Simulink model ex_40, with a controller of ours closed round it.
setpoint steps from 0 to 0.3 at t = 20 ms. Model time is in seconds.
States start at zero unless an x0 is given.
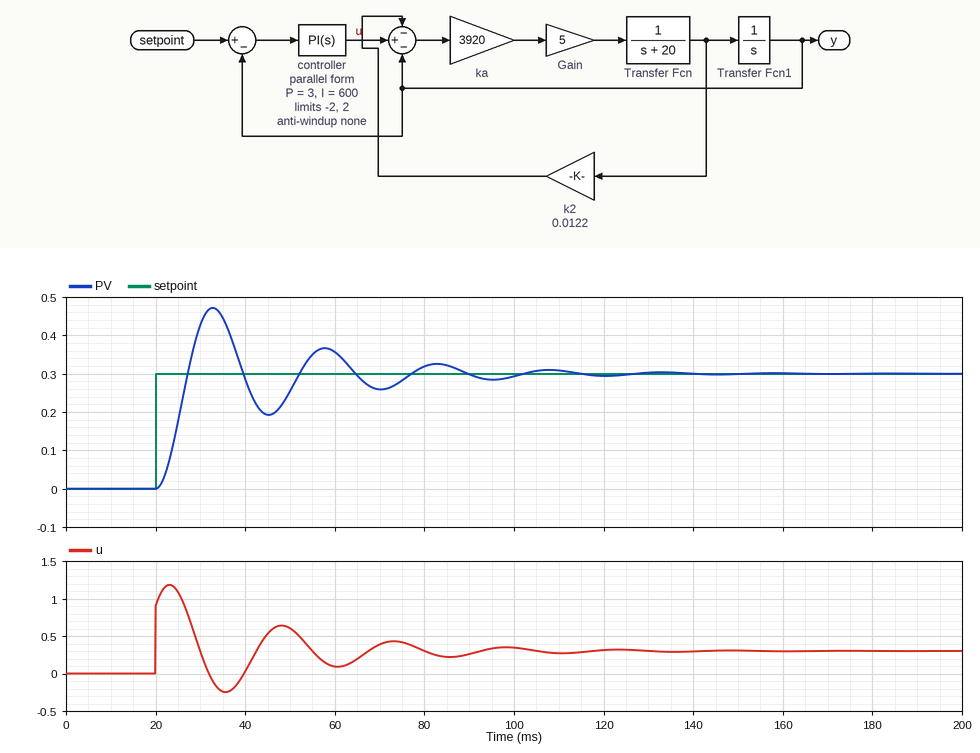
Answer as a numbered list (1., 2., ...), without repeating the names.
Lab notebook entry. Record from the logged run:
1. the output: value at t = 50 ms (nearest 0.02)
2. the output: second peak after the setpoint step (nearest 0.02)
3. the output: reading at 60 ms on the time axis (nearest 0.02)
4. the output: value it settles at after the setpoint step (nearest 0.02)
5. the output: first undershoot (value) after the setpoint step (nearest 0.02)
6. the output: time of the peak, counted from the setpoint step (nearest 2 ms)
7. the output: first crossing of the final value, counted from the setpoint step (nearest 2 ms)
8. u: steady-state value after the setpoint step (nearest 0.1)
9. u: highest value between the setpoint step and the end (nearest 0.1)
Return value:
1. 0.26
2. 0.36
3. 0.36
4. 0.30
5. 0.20
6. 12 ms
7. 8 ms
8. 0.3
9. 1.2
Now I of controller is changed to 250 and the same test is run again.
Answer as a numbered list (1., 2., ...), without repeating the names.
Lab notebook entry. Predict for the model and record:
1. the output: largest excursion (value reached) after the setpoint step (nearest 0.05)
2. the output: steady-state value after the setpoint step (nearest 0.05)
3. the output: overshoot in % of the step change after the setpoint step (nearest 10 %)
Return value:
1. 0.35
2. 0.30
3. 20 %
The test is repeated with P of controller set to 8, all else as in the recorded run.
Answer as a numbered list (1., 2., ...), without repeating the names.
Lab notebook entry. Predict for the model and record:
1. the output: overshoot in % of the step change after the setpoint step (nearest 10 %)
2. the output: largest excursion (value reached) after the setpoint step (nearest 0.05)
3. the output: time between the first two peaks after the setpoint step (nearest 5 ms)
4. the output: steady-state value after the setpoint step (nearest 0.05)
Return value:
1. 40 %
2. 0.45
3. 15 ms
4. 0.30
